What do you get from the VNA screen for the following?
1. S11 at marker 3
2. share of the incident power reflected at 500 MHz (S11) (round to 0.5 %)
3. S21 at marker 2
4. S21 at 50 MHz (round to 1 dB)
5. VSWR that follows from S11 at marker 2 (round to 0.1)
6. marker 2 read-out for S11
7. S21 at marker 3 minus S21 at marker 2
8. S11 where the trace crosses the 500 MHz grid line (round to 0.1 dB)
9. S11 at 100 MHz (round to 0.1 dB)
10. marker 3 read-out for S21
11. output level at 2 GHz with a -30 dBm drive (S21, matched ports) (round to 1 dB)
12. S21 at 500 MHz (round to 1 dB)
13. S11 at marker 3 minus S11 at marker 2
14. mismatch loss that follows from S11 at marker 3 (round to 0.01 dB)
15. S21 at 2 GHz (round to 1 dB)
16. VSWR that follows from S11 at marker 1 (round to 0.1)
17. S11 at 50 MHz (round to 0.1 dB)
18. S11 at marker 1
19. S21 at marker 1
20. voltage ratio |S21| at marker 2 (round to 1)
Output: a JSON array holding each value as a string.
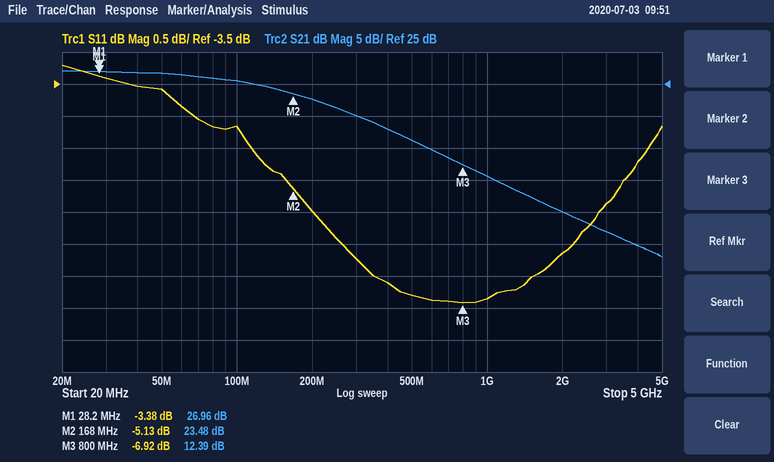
["-6.92 dB", "21.0 %", "23.48 dB", "27 dB", "3.5", "-5.13 dB", "-11.09 dB", "-6.8 dB", "-4.2 dB", "12.39 dB", "-25 dBm", "16 dB", "-1.79 dB", "0.99 dB", "5 dB", "5.2", "-3.6 dB", "-3.38 dB", "26.96 dB", "15"]
